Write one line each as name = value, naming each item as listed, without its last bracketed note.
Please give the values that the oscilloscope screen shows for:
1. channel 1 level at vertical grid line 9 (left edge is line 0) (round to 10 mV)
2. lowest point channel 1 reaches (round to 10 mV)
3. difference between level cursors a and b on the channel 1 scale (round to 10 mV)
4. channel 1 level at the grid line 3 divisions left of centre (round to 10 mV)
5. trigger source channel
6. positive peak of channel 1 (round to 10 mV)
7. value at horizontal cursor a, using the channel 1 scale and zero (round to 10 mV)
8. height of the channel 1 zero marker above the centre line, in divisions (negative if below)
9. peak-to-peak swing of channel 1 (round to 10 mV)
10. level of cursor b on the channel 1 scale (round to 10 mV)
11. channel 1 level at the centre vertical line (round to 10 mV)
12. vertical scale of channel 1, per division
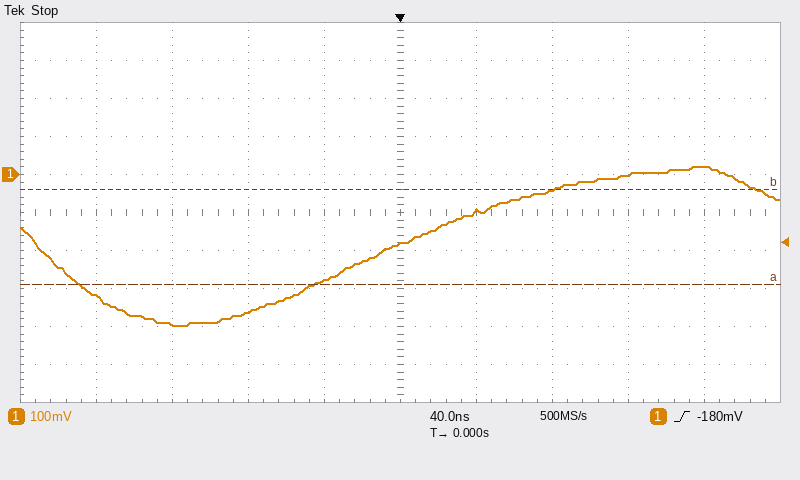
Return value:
channel 1 level at vertical grid line 9 (left edge is line 0) = 20 mV
lowest point channel 1 reaches = -400 mV
difference between level cursors a and b on the channel 1 scale = 250 mV
channel 1 level at the grid line 3 divisions left of centre = -390 mV
trigger source channel = channel 1
positive peak of channel 1 = 20 mV
value at horizontal cursor a, using the channel 1 scale and zero = -290 mV
height of the channel 1 zero marker above the centre line, in divisions = +1.0 div
peak-to-peak swing of channel 1 = 420 mV
level of cursor b on the channel 1 scale = -40 mV
channel 1 level at the centre vertical line = -180 mV
vertical scale of channel 1, per division = 100 mV
